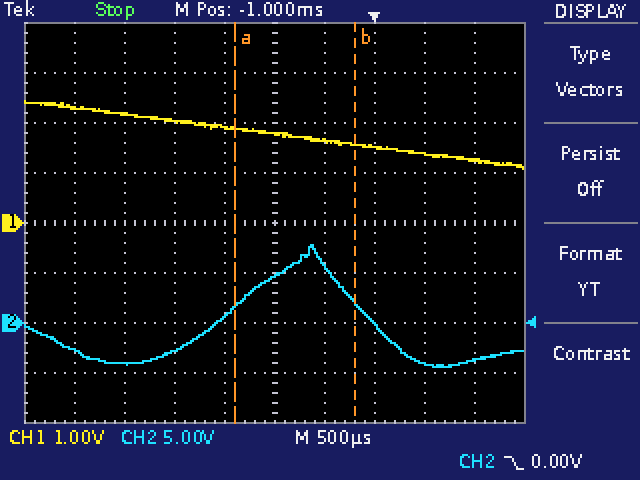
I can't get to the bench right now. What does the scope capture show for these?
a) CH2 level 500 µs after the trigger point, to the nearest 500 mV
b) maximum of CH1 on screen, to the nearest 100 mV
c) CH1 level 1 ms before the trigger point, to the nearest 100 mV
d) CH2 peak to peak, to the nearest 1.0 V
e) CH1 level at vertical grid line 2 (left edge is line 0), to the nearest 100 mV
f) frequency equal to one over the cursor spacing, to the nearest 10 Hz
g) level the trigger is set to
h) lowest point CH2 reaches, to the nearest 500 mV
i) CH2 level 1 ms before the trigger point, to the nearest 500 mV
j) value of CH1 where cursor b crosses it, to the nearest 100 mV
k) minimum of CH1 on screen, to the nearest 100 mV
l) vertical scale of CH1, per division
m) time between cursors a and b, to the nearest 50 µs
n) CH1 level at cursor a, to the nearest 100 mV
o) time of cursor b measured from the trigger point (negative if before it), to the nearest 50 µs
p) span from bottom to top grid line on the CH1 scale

-4.0 V
2.4 V
1.8 V
12.0 V
2.2 V
830 Hz
0.00 V
-4.5 V
4.5 V
1.6 V
1.1 V
1 V
1.20 ms
1.9 V
-200 µs
8 V
